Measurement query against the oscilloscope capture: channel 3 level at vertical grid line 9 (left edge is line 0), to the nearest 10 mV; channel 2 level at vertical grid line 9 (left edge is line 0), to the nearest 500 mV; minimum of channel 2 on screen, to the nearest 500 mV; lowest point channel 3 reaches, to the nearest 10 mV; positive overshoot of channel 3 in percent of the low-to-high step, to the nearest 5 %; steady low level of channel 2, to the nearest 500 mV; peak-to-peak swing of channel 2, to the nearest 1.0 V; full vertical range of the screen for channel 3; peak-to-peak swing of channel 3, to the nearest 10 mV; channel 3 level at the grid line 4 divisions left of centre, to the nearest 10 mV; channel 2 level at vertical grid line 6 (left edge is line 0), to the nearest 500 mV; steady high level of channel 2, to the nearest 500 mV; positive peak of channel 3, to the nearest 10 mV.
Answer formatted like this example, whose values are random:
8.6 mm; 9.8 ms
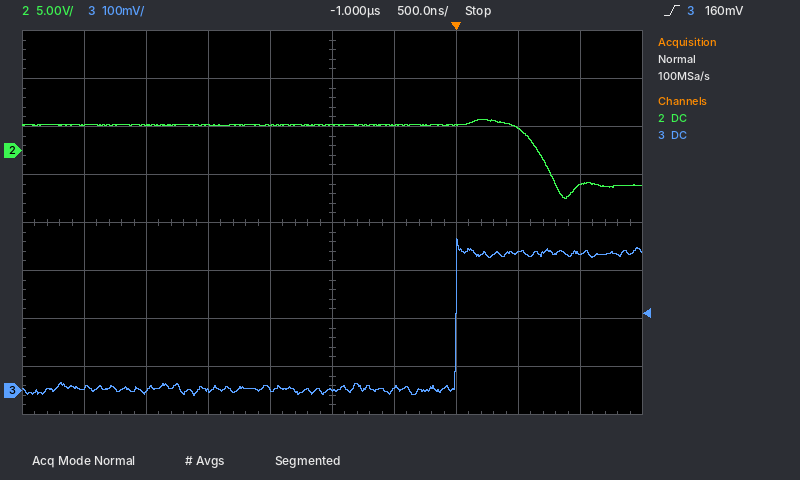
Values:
290 mV; -3.5 V; -5.0 V; -10 mV; 10 %; -3.5 V; 8.0 V; 800 mV; 330 mV; 10 mV; 2.5 V; 2.5 V; 320 mV
